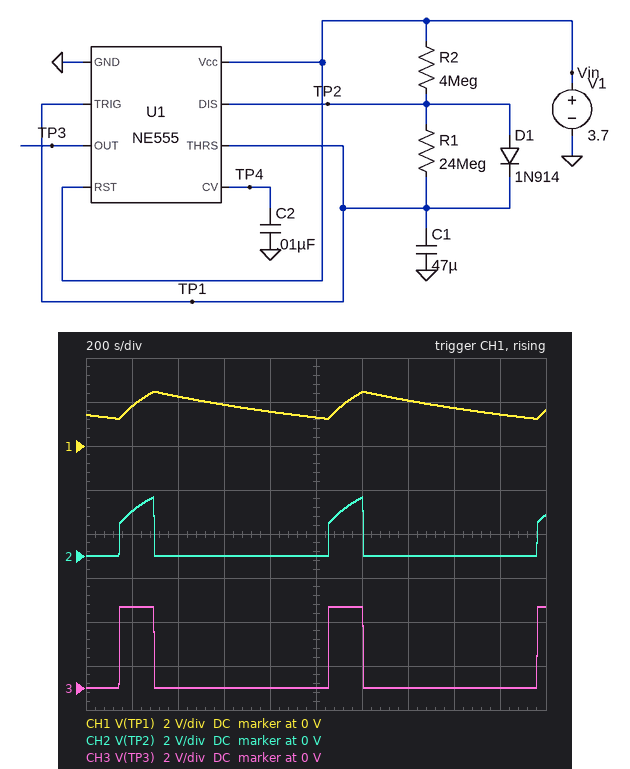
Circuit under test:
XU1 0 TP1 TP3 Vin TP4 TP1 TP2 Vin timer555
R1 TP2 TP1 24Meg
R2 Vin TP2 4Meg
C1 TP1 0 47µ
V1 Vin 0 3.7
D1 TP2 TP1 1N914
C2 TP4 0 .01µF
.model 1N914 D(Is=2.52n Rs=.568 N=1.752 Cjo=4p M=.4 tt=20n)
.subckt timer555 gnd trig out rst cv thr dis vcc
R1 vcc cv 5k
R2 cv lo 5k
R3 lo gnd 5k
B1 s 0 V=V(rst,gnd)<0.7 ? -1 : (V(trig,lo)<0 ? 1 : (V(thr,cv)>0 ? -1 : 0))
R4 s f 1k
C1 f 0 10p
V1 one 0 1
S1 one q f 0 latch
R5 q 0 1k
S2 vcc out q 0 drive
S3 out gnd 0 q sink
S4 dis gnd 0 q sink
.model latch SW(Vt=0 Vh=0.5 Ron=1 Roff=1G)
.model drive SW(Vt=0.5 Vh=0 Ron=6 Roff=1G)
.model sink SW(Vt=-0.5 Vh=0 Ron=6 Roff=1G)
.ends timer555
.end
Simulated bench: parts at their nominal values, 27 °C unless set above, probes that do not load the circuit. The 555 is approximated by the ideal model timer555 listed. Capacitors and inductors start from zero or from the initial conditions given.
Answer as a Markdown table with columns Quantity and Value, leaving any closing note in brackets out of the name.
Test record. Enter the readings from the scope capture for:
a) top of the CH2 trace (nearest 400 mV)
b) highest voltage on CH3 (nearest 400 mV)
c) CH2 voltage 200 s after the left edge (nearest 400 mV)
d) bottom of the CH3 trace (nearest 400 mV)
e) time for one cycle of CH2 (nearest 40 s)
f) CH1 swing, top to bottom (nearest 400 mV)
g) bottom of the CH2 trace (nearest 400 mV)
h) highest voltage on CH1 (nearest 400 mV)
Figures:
| Quantity | Value |
|---|---|
| top of the CH2 trace | 2.8 V |
| highest voltage on CH3 | 3.6 V |
| CH2 voltage 200 s after the left edge | 2.0 V |
| bottom of the CH3 trace | 0 V |
| time for one cycle of CH2 | 920 s |
| CH1 swing, top to bottom | 1.2 V |
| bottom of the CH2 trace | 0 V |
| highest voltage on CH1 | 2.4 V |
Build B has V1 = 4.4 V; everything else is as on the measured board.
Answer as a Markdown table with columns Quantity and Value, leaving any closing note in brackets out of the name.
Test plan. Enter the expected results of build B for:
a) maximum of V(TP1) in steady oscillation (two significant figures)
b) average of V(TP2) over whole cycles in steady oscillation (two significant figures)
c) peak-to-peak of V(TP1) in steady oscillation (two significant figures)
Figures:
| Quantity | Value |
|---|---|
| maximum of V(TP1) in steady oscillation | 2.9 V |
| average of V(TP2) over whole cycles in steady oscillation | 410 mV |
| peak-to-peak of V(TP1) in steady oscillation | 1.5 V |
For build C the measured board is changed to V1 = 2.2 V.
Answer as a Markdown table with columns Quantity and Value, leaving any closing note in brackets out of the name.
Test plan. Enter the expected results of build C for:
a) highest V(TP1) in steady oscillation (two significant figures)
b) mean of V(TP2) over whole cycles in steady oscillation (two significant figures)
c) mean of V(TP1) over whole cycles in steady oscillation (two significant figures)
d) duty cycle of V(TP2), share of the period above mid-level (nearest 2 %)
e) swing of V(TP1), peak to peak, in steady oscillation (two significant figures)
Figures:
| Quantity | Value |
|---|---|
| highest V(TP1) in steady oscillation | 1.5 V |
| mean of V(TP2) over whole cycles in steady oscillation | 240 mV |
| mean of V(TP1) over whole cycles in steady oscillation | 1.1 V |
| duty cycle of V(TP2), share of the period above mid-level | 18 % |
| swing of V(TP1), peak to peak, in steady oscillation | 730 mV |
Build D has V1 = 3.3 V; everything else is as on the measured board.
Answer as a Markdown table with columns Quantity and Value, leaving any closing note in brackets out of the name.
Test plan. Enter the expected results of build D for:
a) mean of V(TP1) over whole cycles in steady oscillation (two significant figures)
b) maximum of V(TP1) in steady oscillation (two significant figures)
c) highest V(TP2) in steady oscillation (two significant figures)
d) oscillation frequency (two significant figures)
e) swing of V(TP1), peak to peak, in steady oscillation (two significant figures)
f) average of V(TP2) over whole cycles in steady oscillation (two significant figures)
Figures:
| Quantity | Value |
|---|---|
| mean of V(TP1) over whole cycles in steady oscillation | 1.6 V |
| maximum of V(TP1) in steady oscillation | 2.2 V |
| highest V(TP2) in steady oscillation | 2.4 V |
| oscillation frequency | 1.1 mHz |
| swing of V(TP1), peak to peak, in steady oscillation | 1.1 V |
| average of V(TP2) over whole cycles in steady oscillation | 330 mV |
